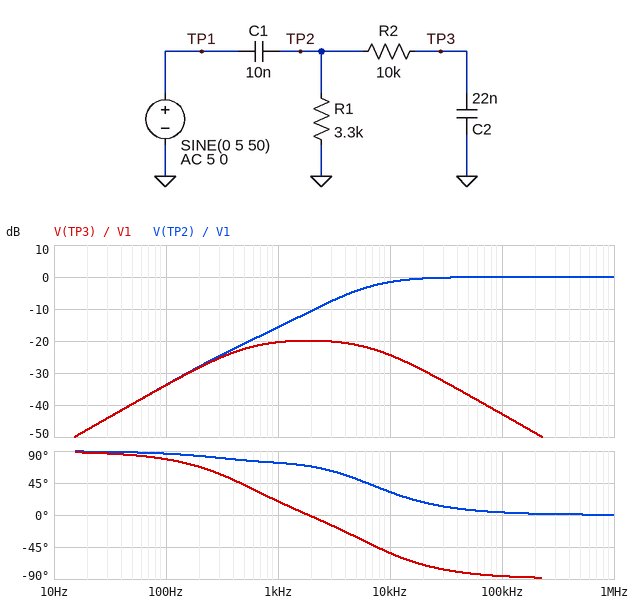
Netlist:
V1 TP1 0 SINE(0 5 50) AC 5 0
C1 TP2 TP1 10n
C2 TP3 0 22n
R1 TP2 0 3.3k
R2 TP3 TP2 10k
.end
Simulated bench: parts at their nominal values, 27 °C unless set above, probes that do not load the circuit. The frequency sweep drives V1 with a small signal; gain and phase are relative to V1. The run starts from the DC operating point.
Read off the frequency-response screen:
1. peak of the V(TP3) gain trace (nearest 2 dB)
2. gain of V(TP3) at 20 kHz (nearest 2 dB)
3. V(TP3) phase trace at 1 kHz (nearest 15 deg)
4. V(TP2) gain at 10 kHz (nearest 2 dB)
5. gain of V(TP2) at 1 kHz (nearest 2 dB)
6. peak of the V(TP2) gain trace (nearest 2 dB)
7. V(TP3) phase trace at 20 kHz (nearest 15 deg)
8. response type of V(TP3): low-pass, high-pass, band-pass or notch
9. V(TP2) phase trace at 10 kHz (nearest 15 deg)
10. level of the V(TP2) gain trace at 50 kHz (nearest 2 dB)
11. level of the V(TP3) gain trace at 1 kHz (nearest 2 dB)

-20 dB
-30 dB
15 deg
-2 dB
-16 dB
0 dB
-75 deg
band-pass
30 deg
0 dB
-20 dB
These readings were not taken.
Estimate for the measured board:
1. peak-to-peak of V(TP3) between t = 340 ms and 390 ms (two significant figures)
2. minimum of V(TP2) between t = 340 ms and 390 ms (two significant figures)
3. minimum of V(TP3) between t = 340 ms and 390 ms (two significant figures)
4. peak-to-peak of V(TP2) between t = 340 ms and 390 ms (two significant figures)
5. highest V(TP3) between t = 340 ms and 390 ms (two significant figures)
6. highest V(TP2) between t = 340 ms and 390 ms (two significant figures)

100 mV
-52 mV
-52 mV
100 mV
52 mV
52 mV
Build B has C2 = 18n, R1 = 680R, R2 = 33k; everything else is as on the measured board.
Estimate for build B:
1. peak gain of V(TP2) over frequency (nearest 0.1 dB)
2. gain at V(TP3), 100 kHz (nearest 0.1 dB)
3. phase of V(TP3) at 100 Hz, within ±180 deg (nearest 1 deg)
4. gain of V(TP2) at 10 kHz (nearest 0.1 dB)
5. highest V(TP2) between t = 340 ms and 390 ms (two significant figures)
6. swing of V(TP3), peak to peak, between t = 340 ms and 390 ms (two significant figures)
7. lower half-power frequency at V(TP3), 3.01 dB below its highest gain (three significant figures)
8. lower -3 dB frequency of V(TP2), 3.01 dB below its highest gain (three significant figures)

0 dB
-51.7 dB
69 deg
-8.3 dB
11 mV
21 mV
257 Hz
23.9 kHz
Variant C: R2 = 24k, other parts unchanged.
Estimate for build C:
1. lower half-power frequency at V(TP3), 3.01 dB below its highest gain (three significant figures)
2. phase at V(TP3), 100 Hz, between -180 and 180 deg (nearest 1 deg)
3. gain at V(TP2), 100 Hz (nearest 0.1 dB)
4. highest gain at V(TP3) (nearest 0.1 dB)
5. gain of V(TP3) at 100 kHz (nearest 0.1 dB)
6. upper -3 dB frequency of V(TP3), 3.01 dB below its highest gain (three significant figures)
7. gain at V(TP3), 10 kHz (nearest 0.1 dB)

241 Hz
68 deg
-33.8 dB
-25.7 dB
-50.4 dB
6.03 kHz
-31.6 dB
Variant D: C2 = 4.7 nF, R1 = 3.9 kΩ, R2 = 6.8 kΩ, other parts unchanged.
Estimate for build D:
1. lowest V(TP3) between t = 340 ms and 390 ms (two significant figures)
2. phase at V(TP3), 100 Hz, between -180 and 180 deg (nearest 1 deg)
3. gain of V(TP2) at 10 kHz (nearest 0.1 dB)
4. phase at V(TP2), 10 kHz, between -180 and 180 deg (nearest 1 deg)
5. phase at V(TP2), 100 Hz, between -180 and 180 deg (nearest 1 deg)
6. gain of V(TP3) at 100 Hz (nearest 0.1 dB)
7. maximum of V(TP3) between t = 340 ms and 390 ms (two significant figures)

-61 mV
87 deg
-1.9 dB
29 deg
88 deg
-32.2 dB
61 mV
